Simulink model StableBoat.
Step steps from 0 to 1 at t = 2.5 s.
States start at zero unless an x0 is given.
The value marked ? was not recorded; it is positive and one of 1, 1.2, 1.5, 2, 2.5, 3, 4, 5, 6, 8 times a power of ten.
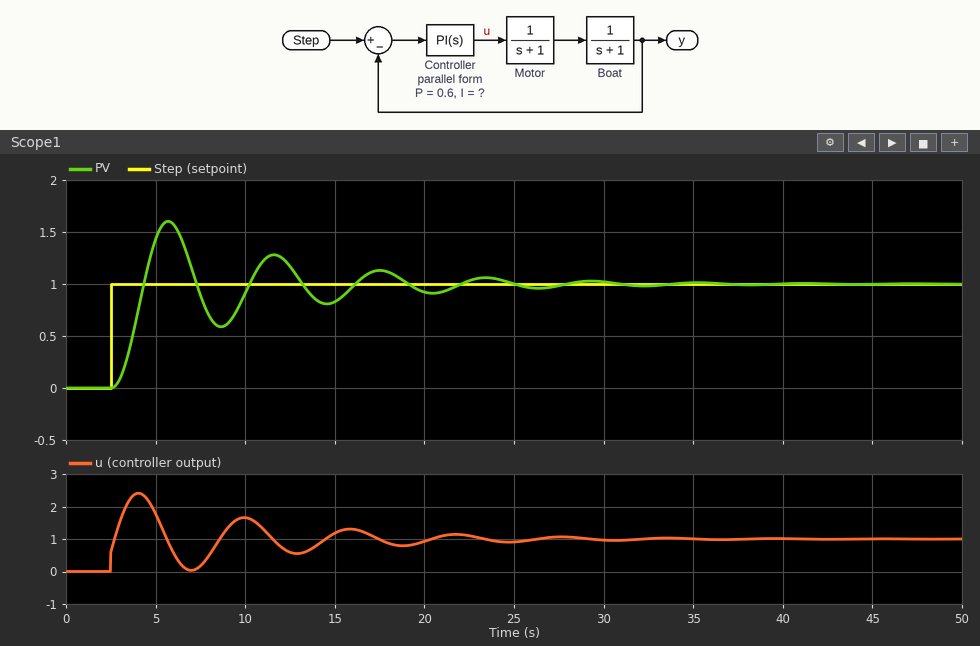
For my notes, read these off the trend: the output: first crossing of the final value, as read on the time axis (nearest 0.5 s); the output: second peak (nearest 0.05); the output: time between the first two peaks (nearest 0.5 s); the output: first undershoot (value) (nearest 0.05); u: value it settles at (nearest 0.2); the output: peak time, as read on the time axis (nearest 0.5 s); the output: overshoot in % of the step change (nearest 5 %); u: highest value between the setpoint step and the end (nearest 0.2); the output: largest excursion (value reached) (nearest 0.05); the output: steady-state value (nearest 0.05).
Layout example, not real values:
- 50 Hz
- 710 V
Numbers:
- 4.5 s
- 1.30
- 6.0 s
- 0.60
- 1.0
- 5.5 s
- 60 %
- 2.4
- 1.60
- 1.00
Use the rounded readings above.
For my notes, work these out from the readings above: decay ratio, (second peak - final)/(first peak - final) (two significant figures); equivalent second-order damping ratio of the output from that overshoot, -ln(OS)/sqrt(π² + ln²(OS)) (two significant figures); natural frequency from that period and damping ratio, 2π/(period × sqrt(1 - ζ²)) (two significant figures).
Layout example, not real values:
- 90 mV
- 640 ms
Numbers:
- 0.50
- 0.16
- 1.1 rad/s
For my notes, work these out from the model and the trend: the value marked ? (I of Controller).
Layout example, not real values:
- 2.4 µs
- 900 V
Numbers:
- 2
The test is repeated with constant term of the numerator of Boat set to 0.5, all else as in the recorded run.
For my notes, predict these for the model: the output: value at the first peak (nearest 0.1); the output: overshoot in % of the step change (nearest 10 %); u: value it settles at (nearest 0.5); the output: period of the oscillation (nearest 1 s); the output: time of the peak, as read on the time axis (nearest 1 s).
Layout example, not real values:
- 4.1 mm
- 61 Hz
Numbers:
- 1.4
- 40 %
- 2.0
- 8 s
- 7 s
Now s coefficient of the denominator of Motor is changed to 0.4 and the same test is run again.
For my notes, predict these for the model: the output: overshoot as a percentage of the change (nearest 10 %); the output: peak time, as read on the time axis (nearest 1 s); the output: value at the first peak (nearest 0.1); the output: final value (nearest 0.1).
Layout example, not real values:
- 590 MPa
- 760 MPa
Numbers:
- 40 %
- 5 s
- 1.4
- 1.0
